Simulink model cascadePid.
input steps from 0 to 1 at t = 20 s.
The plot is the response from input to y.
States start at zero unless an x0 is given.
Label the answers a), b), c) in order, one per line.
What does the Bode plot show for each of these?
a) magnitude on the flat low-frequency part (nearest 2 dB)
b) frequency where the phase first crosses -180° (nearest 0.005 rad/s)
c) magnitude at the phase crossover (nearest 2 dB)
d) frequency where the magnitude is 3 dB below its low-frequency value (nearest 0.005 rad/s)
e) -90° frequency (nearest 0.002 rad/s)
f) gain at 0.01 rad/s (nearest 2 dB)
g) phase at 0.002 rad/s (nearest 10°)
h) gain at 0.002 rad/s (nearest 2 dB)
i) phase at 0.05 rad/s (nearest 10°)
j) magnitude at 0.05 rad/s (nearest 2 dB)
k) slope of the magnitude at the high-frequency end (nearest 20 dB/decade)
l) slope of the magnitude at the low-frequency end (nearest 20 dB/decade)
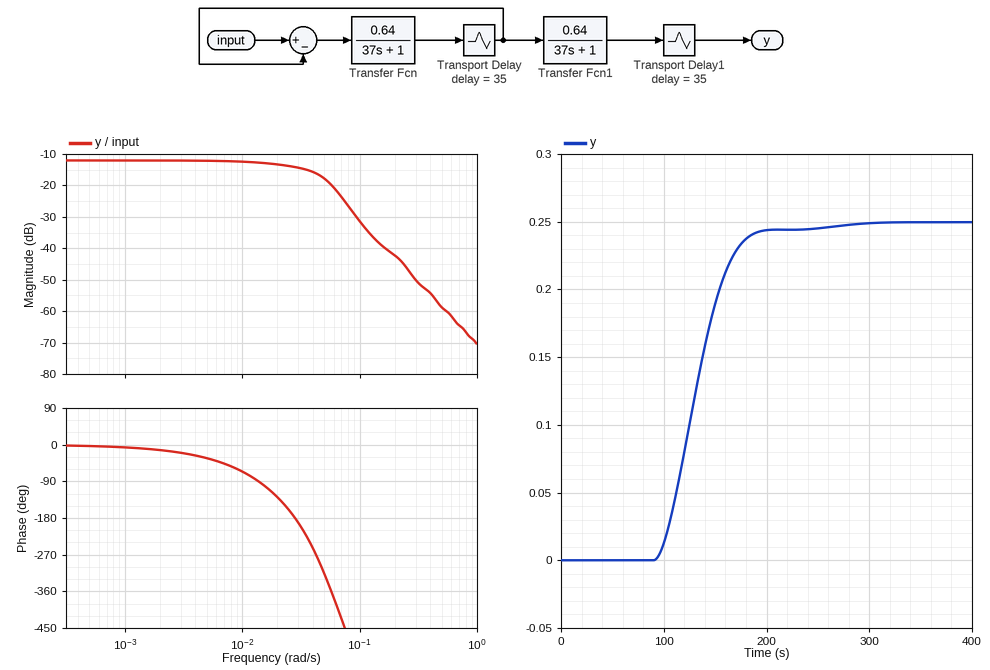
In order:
a) -12 dB
b) 0.030 rad/s
c) -14 dB
d) 0.035 rad/s
e) 0.014 rad/s
f) -12 dB
g) -10°
h) -12 dB
i) -320°
j) -18 dB
k) -40 dB/decade
l) 0 dB/decade
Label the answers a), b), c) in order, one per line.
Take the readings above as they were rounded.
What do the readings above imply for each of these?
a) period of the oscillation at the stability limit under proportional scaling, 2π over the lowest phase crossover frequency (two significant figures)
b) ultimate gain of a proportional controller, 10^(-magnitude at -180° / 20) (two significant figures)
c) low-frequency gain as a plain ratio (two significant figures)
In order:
a) 210 s
b) 5.0
c) 0.25
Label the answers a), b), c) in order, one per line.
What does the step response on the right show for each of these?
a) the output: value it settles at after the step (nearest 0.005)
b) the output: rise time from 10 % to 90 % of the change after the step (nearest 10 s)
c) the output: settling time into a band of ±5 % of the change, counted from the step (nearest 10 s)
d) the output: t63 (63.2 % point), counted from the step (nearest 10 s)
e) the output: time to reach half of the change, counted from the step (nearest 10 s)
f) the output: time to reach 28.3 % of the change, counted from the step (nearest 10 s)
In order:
a) 0.250
b) 60 s
c) 160 s
d) 120 s
e) 110 s
f) 100 s
